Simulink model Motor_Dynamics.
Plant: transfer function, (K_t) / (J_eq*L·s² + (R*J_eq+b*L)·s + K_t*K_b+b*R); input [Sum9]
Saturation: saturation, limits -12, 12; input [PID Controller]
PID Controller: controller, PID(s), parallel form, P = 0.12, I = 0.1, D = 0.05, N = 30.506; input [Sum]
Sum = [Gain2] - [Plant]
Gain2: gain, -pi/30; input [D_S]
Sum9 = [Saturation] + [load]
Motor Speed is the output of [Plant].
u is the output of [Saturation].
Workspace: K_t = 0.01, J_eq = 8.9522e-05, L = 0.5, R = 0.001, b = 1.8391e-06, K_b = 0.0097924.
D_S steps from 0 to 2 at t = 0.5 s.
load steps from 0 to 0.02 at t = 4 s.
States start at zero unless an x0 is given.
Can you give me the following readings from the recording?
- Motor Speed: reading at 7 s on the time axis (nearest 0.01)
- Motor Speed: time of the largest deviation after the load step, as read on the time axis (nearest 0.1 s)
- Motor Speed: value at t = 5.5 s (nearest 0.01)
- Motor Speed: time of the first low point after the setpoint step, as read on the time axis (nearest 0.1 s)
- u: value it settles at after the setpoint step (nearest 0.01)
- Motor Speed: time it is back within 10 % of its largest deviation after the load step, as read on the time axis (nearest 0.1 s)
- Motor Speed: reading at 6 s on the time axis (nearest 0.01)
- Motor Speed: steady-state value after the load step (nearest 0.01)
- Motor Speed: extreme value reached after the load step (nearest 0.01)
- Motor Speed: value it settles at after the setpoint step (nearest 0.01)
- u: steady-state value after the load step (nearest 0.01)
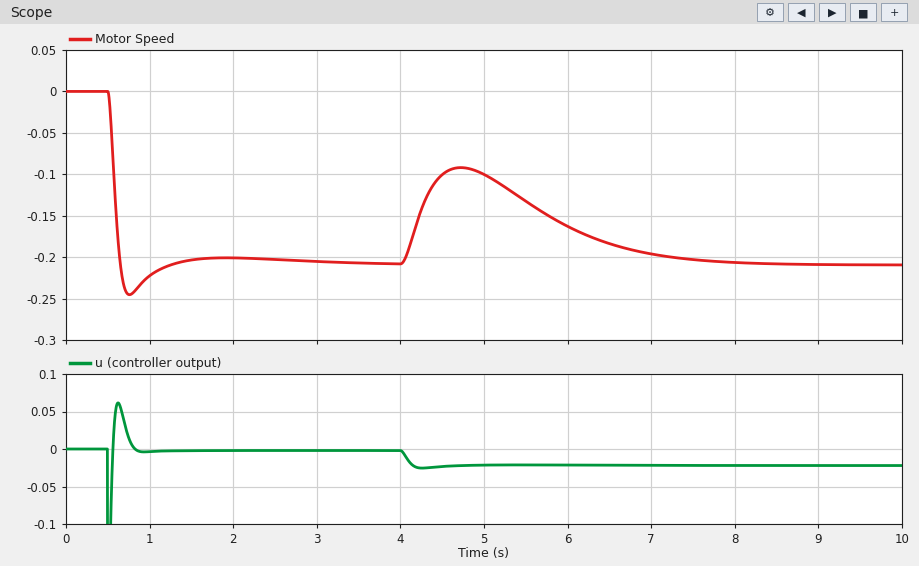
-0.20
4.7 s
-0.13
0.8 s
0.00
7.1 s
-0.16
-0.21
-0.09
-0.21
-0.02
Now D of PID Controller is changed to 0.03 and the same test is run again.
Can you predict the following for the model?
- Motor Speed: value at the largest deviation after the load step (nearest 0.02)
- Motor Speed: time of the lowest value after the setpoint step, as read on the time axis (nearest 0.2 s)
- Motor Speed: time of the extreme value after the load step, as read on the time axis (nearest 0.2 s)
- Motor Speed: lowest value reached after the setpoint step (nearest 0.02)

-0.06
0.8 s
4.6 s
-0.26
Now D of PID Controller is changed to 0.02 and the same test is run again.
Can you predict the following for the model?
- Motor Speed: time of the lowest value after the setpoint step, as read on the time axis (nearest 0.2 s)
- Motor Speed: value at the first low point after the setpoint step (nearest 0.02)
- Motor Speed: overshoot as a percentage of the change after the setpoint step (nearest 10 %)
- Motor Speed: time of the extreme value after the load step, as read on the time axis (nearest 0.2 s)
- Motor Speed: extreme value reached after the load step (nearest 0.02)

1.0 s
-0.30
40 %
4.6 s
-0.04
